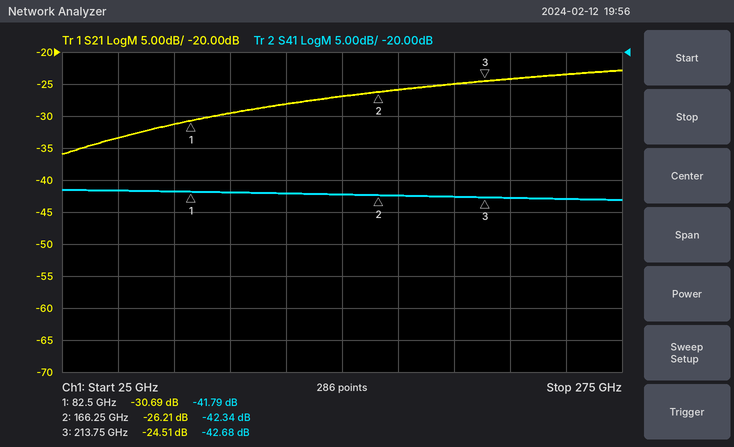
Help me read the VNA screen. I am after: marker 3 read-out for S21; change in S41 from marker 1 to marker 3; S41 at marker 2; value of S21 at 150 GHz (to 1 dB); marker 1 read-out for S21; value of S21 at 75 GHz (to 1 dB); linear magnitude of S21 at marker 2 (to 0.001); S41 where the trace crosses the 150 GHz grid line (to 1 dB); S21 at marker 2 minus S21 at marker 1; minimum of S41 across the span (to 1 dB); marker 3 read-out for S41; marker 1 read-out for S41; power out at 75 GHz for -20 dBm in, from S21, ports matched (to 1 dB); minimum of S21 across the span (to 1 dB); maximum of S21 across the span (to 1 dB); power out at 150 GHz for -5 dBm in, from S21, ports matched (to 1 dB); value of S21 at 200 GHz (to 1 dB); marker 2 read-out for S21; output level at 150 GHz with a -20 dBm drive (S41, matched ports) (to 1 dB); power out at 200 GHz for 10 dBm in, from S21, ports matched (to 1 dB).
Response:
-24.51 dB
-0.89 dB
-42.34 dB
-27 dB
-30.69 dB
-31 dB
0.049
-42 dB
4.48 dB
-43 dB
-42.68 dB
-41.79 dB
-51 dBm
-36 dB
-23 dB
-32 dBm
-25 dB
-26.21 dB
-62 dBm
-15 dBm
